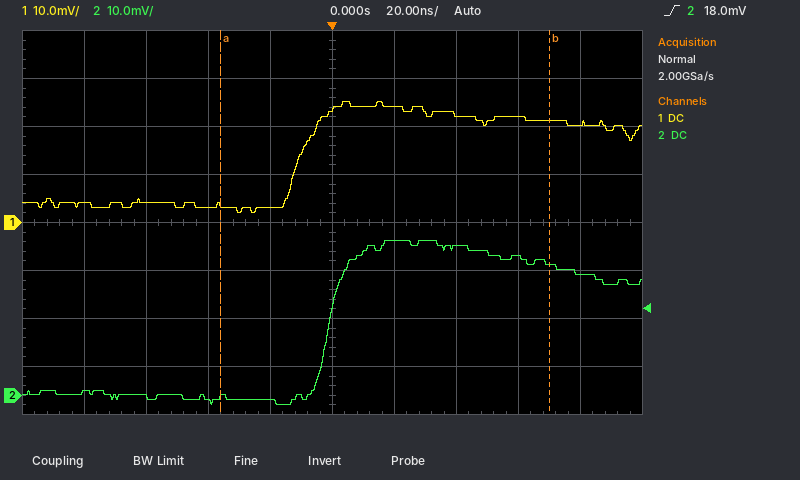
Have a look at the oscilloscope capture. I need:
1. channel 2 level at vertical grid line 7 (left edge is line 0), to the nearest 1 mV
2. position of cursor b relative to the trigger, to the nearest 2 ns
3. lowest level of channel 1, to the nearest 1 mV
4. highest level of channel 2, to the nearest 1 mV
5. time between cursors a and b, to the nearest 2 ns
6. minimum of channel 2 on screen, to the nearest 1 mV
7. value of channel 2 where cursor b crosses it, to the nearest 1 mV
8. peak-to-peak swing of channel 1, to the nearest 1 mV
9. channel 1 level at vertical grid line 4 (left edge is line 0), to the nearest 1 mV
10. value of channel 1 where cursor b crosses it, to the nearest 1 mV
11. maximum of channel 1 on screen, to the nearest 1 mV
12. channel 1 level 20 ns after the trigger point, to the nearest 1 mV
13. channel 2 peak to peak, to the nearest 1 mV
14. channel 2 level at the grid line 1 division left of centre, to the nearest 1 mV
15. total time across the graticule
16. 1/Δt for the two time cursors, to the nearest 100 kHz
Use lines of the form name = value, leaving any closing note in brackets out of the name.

channel 2 level at vertical grid line 7 (left edge is line 0), to the nearest 1 mV = 31 mV
position of cursor b relative to the trigger, to the nearest 2 ns = +70 ns
lowest level of channel 1, to the nearest 1 mV = 2 mV
highest level of channel 2, to the nearest 1 mV = 32 mV
time between cursors a and b, to the nearest 2 ns = 106 ns
minimum of channel 2 on screen, to the nearest 1 mV = -2 mV
value of channel 2 where cursor b crosses it, to the nearest 1 mV = 27 mV
peak-to-peak swing of channel 1, to the nearest 1 mV = 23 mV
channel 1 level at vertical grid line 4 (left edge is line 0), to the nearest 1 mV = 3 mV
value of channel 1 where cursor b crosses it, to the nearest 1 mV = 21 mV
maximum of channel 1 on screen, to the nearest 1 mV = 25 mV
channel 1 level 20 ns after the trigger point, to the nearest 1 mV = 24 mV
channel 2 peak to peak, to the nearest 1 mV = 34 mV
channel 2 level at the grid line 1 division left of centre, to the nearest 1 mV = -1 mV
total time across the graticule = 200 ns
1/Δt for the two time cursors, to the nearest 100 kHz = 9.4 MHz
